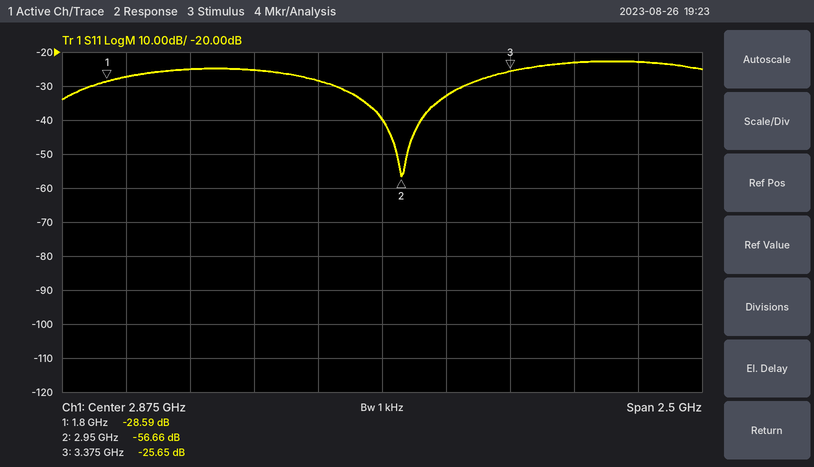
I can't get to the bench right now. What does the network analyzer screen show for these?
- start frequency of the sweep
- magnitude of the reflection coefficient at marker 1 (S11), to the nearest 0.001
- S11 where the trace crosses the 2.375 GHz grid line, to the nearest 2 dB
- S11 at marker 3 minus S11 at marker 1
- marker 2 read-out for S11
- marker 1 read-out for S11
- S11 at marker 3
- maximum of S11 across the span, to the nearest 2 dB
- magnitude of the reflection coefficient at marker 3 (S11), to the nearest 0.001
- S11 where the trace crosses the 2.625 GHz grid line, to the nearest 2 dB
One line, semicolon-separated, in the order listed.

1.625 GHz; 0.037; -26 dB; 2.94 dB; -56.66 dB; -28.59 dB; -25.65 dB; -22 dB; 0.052; -28 dB
